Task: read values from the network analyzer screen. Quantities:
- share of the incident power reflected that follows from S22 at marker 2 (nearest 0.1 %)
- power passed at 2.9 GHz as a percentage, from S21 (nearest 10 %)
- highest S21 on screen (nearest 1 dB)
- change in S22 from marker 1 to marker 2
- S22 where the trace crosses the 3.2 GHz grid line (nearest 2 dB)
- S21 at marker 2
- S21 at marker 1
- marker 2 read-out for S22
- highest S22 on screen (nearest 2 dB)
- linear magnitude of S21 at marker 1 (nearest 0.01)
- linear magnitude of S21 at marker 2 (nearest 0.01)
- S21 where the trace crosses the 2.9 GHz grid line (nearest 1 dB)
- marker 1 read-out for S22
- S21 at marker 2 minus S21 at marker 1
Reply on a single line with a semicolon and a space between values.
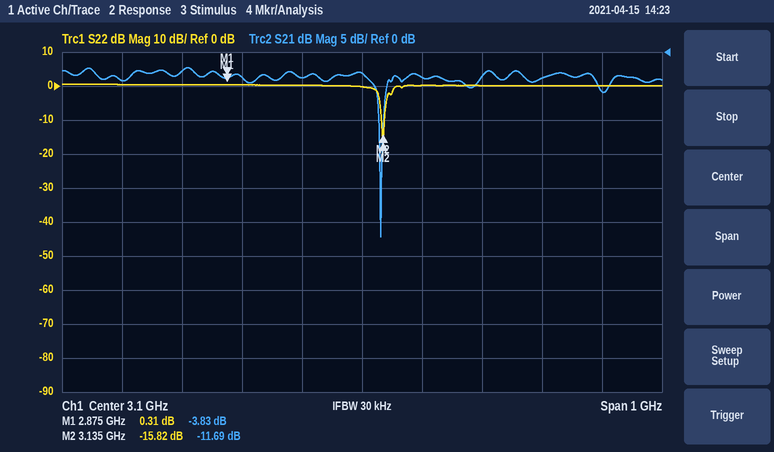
2.6 %; 40 %; -2 dB; -16.13 dB; 0 dB; -11.69 dB; -3.83 dB; -15.82 dB; 0 dB; 0.64; 0.26; -4 dB; 0.31 dB; -7.86 dB
